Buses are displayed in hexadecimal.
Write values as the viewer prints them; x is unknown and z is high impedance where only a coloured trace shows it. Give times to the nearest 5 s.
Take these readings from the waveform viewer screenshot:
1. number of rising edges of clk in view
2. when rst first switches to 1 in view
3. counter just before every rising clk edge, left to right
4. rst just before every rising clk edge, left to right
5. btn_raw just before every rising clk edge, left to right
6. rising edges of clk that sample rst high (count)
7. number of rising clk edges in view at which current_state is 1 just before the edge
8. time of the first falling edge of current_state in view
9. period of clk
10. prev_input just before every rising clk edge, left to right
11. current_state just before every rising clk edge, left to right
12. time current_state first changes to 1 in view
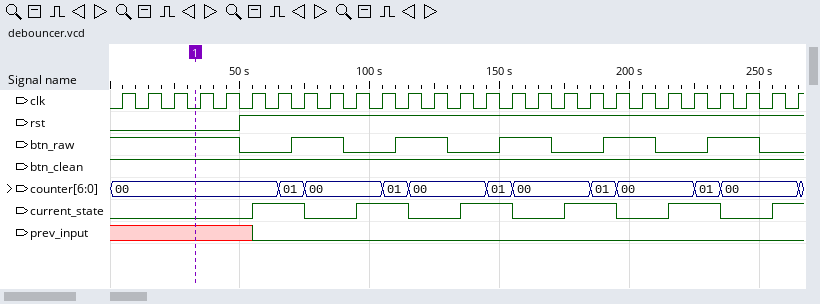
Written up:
27
50 s
00, 00, 00, 00, 00, 00, 00, 01, 00, 00, 00, 01, 00, 00, 00, 01, 00, 00, 00, 01, 00, 00, 00, 01, 00, 00, 00
0 0 0 0 0 1 1 1 1 1 1 1 1 1 1 1 1 1 1 1 1 1 1 1 1 1 1
1 1 1 1 1 0 0 1 1 0 0 1 1 0 0 1 1 0 0 1 1 0 0 1 1 0 0
22
11
75 s
10 s
x x x x x x 0 0 0 0 0 0 0 0 0 0 0 0 0 0 0 0 0 0 0 0 0
0 0 0 0 0 0 1 1 0 0 1 1 0 0 1 1 0 0 1 1 0 0 1 1 0 0 1
55 s
